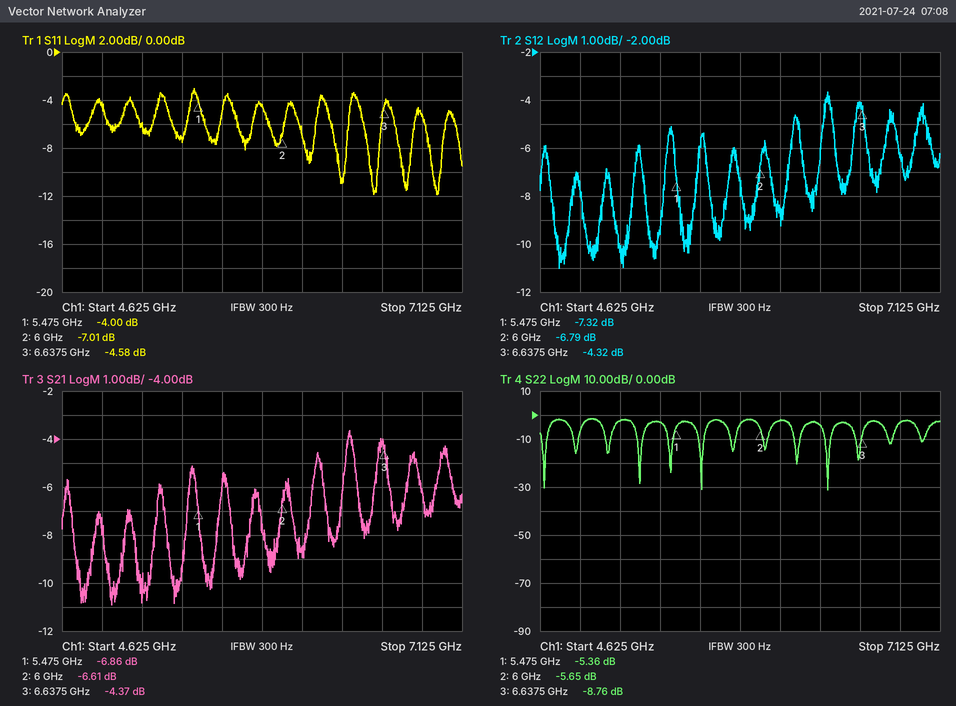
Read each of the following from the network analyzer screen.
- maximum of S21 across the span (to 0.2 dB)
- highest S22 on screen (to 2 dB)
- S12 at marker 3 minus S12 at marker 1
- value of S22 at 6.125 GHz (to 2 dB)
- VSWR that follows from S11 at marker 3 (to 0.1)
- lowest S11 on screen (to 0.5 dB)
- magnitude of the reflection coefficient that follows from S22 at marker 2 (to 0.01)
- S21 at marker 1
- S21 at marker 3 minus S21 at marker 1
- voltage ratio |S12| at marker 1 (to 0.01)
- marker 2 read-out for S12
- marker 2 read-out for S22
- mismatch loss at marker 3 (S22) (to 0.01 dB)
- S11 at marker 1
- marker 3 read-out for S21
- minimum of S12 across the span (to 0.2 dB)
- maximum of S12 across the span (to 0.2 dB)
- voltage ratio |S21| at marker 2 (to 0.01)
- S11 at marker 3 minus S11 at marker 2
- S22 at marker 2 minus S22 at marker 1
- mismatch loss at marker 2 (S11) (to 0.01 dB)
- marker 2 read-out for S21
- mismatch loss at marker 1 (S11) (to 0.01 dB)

-3.6 dB
-2 dB
3.00 dB
-2 dB
3.9
-12.0 dB
0.52
-6.86 dB
2.49 dB
0.43
-6.79 dB
-5.65 dB
0.62 dB
-4.00 dB
-4.37 dB
-11.0 dB
-3.6 dB
0.47
2.43 dB
-0.29 dB
0.96 dB
-6.61 dB
2.20 dB
